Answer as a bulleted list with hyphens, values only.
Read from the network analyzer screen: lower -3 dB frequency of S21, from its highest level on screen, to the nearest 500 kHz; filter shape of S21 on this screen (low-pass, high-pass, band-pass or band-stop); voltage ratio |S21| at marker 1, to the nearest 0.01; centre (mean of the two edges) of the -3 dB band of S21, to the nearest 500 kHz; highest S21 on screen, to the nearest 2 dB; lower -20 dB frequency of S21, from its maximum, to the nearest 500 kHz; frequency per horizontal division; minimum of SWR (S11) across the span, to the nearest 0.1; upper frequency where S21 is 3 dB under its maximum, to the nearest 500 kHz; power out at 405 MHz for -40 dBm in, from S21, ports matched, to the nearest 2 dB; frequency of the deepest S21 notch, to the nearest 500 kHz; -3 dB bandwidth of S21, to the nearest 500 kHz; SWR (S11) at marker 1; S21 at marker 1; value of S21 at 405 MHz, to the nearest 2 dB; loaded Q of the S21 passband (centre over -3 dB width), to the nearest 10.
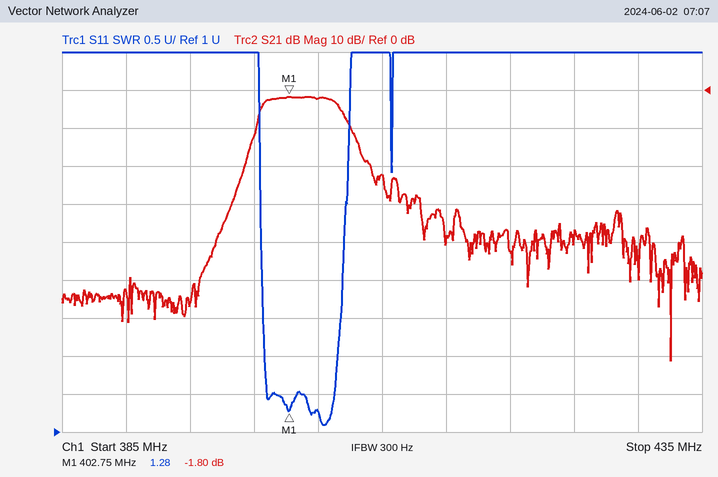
- 400.5 MHz
- band-pass
- 0.81
- 403.5 MHz
- -2 dB
- 399.0 MHz
- 5 MHz
- 1.1
- 406.5 MHz
- -42 dBm
- 432.5 MHz
- 6.0 MHz
- 1.28
- -1.80 dB
- -2 dB
- 70
